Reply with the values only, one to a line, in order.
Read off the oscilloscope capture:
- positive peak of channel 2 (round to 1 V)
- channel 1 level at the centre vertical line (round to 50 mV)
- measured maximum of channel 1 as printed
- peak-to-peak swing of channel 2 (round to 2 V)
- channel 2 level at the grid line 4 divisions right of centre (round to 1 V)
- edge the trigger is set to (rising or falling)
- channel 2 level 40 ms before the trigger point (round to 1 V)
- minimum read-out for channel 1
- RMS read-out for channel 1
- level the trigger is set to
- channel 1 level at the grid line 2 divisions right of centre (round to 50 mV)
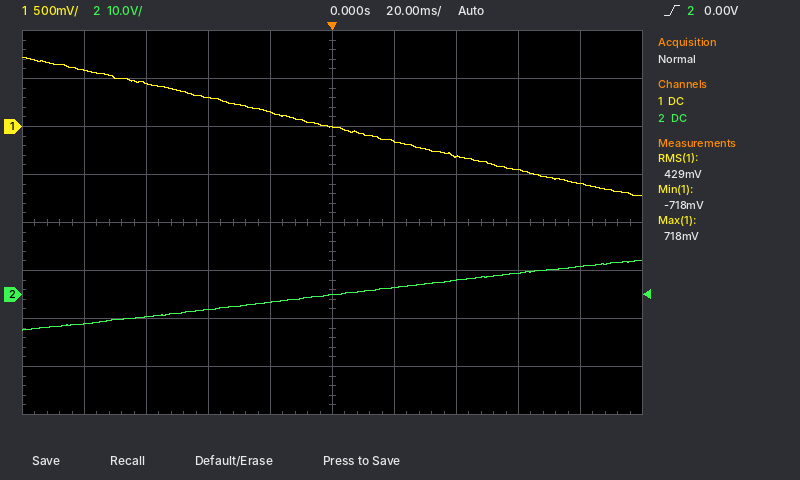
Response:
7 V
0 mV
718 mV
14 V
6 V
rising
-3 V
-718 mV
429 mV
0.00 V
-300 mV
